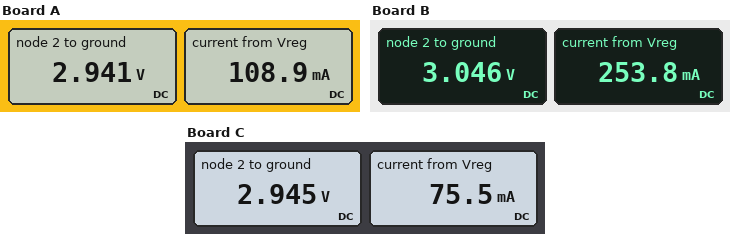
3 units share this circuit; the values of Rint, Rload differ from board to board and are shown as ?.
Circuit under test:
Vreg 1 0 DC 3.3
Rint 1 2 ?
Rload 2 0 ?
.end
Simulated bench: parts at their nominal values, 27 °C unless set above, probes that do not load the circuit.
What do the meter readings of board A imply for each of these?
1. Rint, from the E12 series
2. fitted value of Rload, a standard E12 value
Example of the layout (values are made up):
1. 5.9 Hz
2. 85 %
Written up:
1. 3.3 Ω
2. 27 Ω
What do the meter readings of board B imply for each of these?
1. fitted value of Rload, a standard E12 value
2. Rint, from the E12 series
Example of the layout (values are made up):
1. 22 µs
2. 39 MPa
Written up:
1. 12 Ω
2. 1 Ω
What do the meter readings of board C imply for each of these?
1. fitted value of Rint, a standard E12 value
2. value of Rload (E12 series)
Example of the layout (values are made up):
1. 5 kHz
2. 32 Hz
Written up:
1. 4.7 Ω
2. 39 Ω
